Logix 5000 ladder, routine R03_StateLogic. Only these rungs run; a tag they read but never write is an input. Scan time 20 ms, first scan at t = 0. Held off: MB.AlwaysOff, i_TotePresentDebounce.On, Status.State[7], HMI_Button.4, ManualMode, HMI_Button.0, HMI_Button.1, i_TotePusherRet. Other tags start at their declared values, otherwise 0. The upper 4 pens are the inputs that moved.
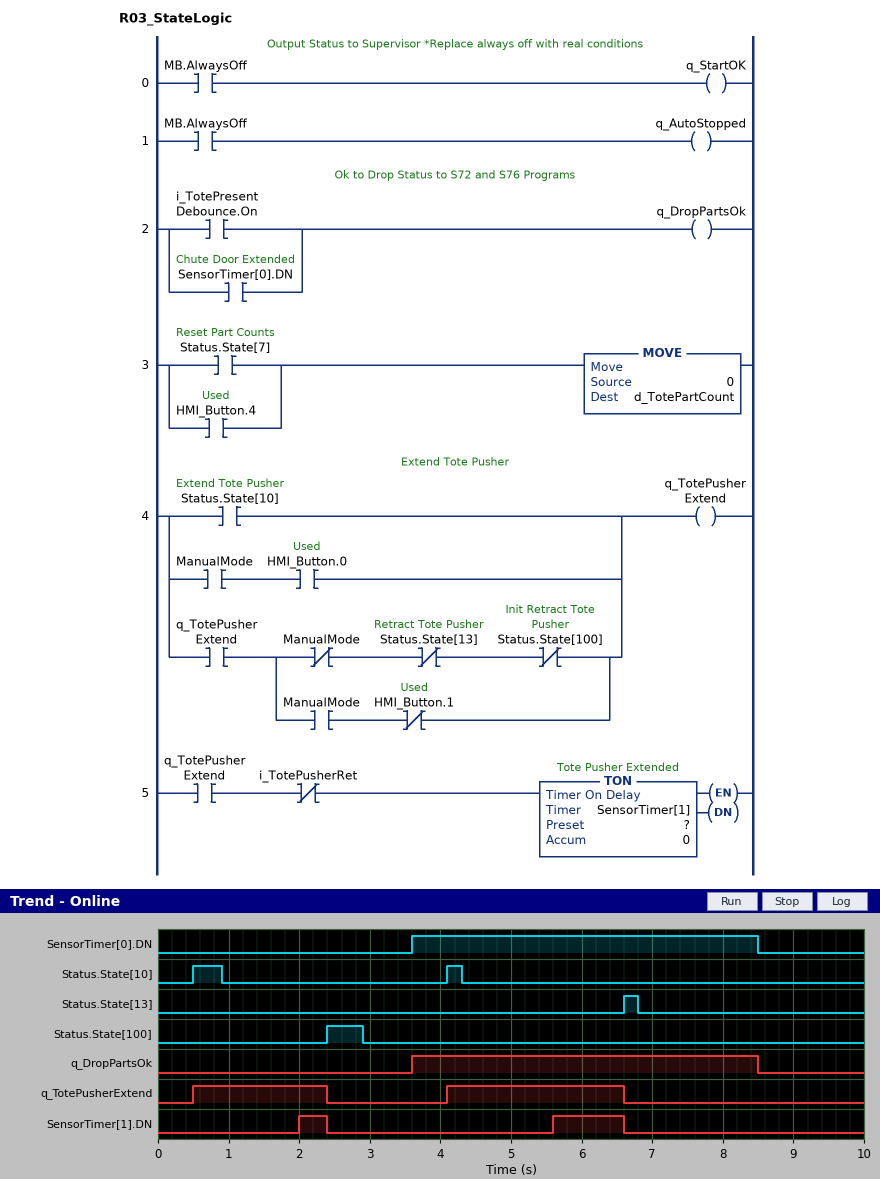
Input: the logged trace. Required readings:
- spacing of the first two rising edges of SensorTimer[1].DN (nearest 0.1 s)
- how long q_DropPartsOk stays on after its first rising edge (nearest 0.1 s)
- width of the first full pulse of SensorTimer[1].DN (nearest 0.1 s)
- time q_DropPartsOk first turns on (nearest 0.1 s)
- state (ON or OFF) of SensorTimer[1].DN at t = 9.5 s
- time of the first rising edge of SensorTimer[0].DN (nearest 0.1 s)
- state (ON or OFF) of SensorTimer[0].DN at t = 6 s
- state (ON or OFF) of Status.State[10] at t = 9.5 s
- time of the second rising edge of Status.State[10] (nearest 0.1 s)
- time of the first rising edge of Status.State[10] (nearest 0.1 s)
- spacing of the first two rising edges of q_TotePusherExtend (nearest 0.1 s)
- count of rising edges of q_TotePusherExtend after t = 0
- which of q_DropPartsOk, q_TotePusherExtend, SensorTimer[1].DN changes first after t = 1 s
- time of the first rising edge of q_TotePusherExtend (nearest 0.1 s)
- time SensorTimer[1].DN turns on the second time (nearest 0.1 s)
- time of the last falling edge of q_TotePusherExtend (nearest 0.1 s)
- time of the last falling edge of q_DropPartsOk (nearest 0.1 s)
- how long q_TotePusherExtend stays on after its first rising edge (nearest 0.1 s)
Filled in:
3.6 s
4.9 s
0.4 s
3.6 s
OFF
3.6 s
ON
OFF
4.1 s
0.5 s
3.6 s
2
SensorTimer[1].DN
0.5 s
5.6 s
6.6 s
8.5 s
1.9 s
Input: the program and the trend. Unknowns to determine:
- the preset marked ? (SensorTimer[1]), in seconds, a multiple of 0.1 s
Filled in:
1.5 s
